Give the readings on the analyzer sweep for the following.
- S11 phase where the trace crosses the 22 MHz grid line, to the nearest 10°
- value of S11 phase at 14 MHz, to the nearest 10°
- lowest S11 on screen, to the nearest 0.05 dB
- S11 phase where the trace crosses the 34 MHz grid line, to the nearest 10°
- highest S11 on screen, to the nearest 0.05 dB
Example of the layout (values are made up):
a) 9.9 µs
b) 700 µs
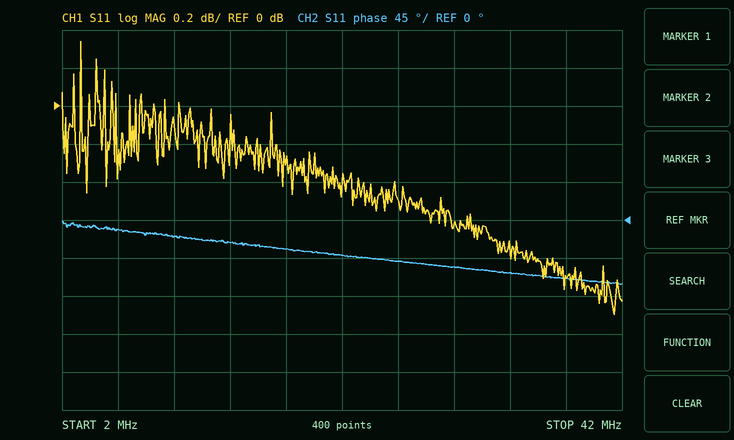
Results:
a) -40°
b) -30°
c) -1.10 dB
d) -60°
e) 0.35 dB
